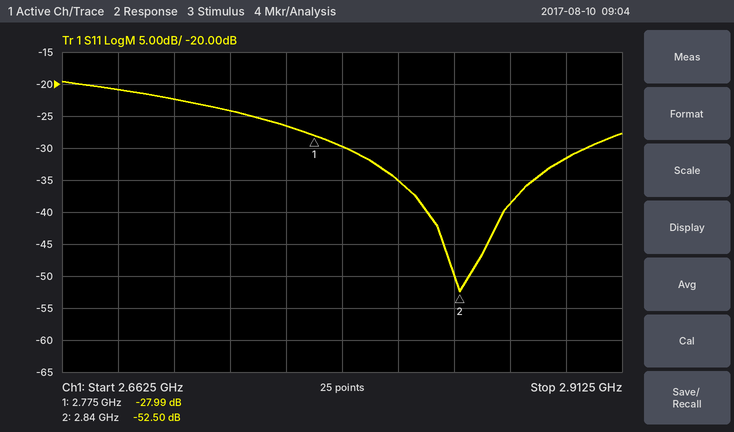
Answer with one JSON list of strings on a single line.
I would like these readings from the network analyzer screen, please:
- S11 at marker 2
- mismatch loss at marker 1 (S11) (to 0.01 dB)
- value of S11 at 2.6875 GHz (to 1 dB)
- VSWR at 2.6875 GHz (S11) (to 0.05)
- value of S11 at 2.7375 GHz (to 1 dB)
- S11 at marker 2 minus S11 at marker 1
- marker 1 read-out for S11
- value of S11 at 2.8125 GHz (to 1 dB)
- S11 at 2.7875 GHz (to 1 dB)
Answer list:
["-52.50 dB", "0.01 dB", "-21 dB", "1.20", "-24 dB", "-24.51 dB", "-27.99 dB", "-35 dB", "-30 dB"]
